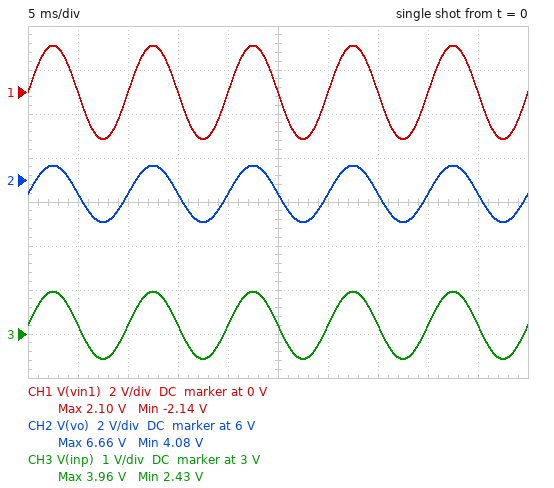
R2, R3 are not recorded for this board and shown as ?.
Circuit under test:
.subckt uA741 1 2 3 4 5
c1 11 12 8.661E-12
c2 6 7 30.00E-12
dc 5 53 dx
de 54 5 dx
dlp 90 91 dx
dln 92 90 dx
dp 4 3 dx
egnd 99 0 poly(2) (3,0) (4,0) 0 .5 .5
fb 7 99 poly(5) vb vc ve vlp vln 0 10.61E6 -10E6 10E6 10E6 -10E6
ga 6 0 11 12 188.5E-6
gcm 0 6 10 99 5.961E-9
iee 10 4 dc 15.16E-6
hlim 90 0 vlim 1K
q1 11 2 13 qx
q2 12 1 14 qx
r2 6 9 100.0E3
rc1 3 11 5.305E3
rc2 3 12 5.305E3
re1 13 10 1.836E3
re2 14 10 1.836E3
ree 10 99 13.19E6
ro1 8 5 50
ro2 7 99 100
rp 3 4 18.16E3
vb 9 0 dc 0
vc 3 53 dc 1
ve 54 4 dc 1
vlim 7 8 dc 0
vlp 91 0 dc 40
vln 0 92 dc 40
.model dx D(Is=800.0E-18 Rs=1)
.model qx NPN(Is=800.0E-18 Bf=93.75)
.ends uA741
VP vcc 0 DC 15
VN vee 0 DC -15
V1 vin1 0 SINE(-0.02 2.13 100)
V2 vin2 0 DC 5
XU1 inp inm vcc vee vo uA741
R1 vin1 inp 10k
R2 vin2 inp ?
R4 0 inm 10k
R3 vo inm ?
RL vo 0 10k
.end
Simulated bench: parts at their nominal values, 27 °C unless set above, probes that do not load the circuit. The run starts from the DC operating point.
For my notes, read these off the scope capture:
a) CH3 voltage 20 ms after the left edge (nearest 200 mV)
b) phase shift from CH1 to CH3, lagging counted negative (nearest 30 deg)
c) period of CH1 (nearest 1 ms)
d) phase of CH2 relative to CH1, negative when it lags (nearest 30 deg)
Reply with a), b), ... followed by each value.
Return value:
a) 3.2 V
b) 0 deg
c) 10 ms
d) 0 deg
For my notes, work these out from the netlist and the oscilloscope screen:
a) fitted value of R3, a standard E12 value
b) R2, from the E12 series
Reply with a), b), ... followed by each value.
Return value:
a) 6.8 kΩ
b) 5.6 kΩ
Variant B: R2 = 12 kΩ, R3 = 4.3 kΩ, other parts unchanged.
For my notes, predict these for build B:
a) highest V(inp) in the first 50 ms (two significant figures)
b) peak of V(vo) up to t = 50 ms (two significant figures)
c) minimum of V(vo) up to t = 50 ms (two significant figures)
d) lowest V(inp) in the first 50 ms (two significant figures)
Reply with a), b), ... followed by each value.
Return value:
a) 3.4 V
b) 4.9 V
c) 1.6 V
d) 1.1 V
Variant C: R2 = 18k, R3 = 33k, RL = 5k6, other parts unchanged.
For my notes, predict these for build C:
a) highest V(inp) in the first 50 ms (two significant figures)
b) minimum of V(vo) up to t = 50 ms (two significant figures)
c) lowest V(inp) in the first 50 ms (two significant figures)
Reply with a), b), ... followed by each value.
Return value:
a) 3.1 V
b) 1.7 V
c) 400 mV
